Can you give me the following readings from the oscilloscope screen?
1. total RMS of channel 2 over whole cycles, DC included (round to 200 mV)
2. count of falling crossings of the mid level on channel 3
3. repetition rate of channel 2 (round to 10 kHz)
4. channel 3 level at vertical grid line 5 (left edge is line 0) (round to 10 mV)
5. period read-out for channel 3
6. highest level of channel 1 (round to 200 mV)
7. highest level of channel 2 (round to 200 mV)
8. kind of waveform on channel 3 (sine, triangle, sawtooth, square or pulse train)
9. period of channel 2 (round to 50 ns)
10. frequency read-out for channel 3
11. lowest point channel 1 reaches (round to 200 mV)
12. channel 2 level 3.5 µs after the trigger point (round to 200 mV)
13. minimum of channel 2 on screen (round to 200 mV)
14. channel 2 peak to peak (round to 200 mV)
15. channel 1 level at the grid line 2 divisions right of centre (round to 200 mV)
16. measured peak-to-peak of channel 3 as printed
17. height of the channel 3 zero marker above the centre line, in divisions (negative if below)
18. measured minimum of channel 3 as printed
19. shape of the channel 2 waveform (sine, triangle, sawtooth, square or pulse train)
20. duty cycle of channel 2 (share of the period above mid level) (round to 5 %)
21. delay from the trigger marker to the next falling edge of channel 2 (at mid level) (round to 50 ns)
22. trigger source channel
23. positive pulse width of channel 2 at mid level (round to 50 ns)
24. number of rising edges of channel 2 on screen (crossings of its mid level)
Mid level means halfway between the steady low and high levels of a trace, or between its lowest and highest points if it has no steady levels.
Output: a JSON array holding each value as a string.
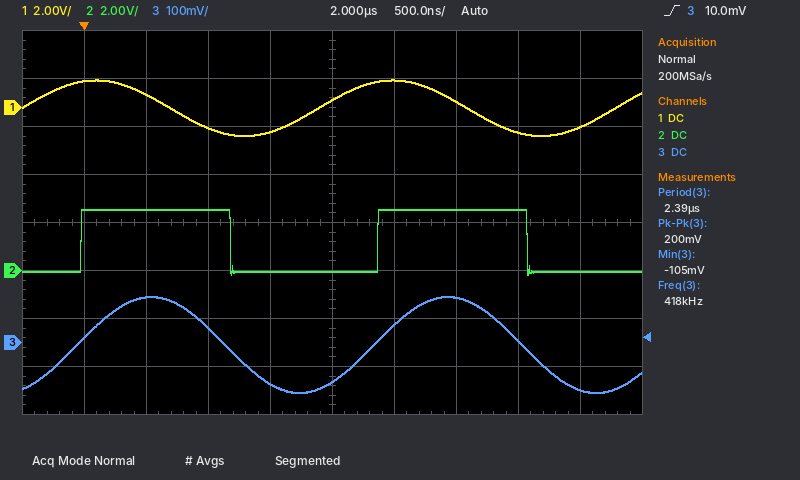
["1.8 V", "2", "420 kHz", "-80 mV", "2.39 µs", "1.2 V", "2.6 V", "sine", "2.40 µs", "418 kHz", "-1.2 V", "2.6 V", "-200 mV", "2.8 V", "200 mV", "200 mV", "-2.5 div", "-105 mV", "square", "50 %", "1.20 µs", "channel 3", "1.20 µs", "2"]
